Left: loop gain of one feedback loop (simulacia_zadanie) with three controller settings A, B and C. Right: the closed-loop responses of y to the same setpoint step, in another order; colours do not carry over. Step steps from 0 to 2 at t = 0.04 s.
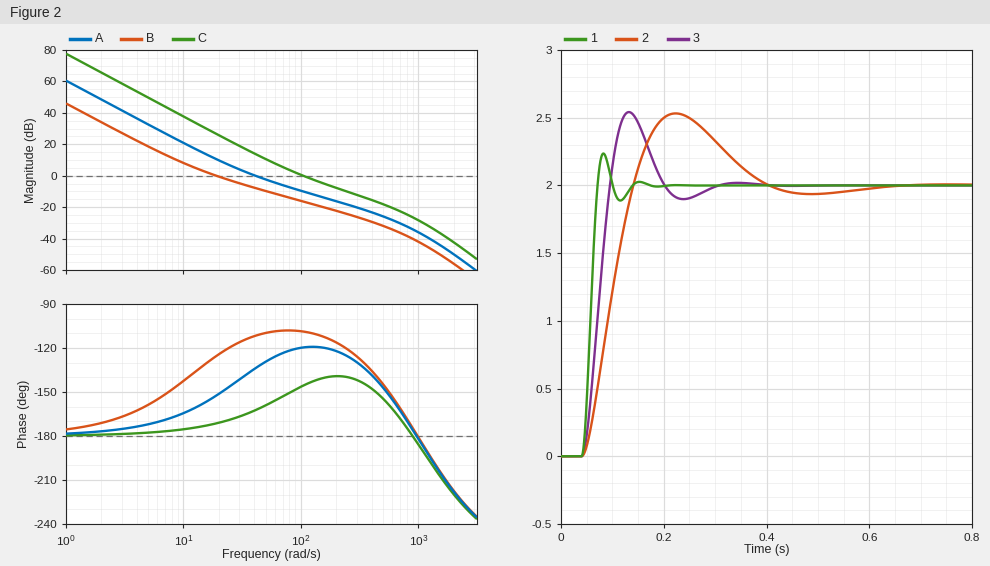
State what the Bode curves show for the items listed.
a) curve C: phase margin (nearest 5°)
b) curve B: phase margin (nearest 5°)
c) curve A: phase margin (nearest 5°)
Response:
35°
55°
45°
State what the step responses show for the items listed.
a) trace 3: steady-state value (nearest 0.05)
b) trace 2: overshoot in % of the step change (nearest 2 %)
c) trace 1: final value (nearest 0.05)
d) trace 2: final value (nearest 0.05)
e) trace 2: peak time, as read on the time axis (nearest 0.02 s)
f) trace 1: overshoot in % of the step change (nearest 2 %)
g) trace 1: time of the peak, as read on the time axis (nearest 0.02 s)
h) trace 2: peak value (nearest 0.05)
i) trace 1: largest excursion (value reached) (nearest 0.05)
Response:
2.00
26 %
2.00
2.00
0.22 s
12 %
0.08 s
2.55
2.25
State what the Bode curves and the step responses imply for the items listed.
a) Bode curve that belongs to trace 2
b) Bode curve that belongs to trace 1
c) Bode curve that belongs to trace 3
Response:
B
C
A
